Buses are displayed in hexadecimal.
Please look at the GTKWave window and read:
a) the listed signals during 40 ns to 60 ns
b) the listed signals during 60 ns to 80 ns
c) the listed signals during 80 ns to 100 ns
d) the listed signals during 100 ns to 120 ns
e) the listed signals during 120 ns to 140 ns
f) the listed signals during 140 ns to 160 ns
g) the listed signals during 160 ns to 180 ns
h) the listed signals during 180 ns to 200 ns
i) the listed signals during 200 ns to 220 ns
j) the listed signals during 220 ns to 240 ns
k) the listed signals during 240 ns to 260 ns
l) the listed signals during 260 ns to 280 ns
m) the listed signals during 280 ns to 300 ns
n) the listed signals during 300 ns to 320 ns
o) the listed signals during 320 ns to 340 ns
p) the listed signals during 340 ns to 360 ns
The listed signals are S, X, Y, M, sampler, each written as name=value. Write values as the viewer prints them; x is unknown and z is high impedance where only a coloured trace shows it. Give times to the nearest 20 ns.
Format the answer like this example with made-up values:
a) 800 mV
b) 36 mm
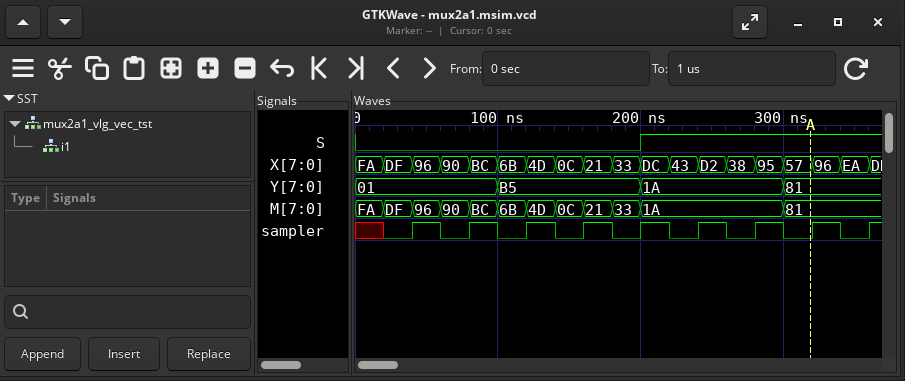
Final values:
a) S=0, X=96, Y=01, M=96, sampler=1
b) S=0, X=90, Y=01, M=90, sampler=0
c) S=0, X=BC, Y=01, M=BC, sampler=1
d) S=0, X=6B, Y=B5, M=6B, sampler=0
e) S=0, X=4D, Y=B5, M=4D, sampler=1
f) S=0, X=0C, Y=B5, M=0C, sampler=0
g) S=0, X=21, Y=B5, M=21, sampler=1
h) S=0, X=33, Y=B5, M=33, sampler=0
i) S=1, X=DC, Y=1A, M=1A, sampler=1
j) S=1, X=43, Y=1A, M=1A, sampler=0
k) S=1, X=D2, Y=1A, M=1A, sampler=1
l) S=1, X=38, Y=1A, M=1A, sampler=0
m) S=1, X=95, Y=1A, M=1A, sampler=1
n) S=1, X=57, Y=81, M=81, sampler=0
o) S=1, X=96, Y=81, M=81, sampler=1
p) S=1, X=EA, Y=81, M=81, sampler=0
